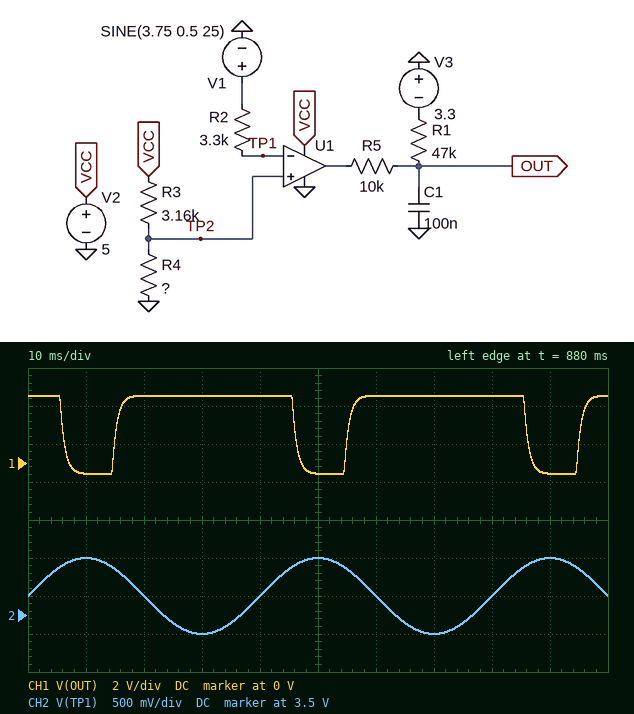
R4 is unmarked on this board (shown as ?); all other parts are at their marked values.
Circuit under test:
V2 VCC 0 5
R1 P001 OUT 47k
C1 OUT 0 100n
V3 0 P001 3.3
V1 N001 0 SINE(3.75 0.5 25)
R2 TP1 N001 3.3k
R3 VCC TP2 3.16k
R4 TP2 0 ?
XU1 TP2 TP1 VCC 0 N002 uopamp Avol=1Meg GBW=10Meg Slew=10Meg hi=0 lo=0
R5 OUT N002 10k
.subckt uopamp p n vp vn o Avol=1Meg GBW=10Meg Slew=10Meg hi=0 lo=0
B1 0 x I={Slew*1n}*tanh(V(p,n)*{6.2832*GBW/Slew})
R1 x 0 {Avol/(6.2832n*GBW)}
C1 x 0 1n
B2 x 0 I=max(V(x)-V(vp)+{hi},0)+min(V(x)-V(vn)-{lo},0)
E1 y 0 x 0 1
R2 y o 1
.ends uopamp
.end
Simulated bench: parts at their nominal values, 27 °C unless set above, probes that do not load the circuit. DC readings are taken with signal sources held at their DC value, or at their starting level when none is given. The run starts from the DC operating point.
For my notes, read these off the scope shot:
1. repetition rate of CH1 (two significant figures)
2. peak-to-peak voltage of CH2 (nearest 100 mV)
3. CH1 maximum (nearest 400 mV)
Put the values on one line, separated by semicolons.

25 Hz; 1.0 V; 3.6 V
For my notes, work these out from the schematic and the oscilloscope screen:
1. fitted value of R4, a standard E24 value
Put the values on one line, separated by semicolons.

15 kΩ
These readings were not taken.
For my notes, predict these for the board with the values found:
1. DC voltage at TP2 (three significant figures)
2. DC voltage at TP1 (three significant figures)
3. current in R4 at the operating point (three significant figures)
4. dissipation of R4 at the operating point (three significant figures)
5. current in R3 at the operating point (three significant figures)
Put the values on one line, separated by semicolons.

4.13 V; 3.75 V; 275 µA; 1.14 mW; 275 µA
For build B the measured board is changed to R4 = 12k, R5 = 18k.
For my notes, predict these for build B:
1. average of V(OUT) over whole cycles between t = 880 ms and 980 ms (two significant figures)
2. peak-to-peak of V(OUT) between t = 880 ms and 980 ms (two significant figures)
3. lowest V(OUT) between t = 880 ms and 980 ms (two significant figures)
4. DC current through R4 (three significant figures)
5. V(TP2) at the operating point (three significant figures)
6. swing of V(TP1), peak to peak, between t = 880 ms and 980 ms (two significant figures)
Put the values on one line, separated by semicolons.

1.4 V; 3.6 V; -920 mV; 330 µA; 3.96 V; 1.0 V
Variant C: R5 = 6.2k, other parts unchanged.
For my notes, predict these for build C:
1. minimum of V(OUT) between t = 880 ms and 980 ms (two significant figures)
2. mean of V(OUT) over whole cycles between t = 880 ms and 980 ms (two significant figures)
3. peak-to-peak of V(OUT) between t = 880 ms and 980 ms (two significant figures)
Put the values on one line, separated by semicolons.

-390 mV; 3.0 V; 4.4 V
